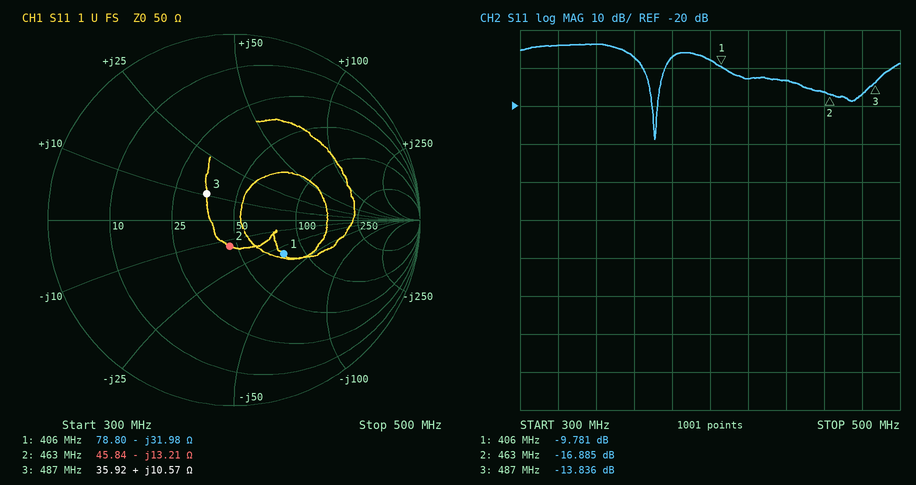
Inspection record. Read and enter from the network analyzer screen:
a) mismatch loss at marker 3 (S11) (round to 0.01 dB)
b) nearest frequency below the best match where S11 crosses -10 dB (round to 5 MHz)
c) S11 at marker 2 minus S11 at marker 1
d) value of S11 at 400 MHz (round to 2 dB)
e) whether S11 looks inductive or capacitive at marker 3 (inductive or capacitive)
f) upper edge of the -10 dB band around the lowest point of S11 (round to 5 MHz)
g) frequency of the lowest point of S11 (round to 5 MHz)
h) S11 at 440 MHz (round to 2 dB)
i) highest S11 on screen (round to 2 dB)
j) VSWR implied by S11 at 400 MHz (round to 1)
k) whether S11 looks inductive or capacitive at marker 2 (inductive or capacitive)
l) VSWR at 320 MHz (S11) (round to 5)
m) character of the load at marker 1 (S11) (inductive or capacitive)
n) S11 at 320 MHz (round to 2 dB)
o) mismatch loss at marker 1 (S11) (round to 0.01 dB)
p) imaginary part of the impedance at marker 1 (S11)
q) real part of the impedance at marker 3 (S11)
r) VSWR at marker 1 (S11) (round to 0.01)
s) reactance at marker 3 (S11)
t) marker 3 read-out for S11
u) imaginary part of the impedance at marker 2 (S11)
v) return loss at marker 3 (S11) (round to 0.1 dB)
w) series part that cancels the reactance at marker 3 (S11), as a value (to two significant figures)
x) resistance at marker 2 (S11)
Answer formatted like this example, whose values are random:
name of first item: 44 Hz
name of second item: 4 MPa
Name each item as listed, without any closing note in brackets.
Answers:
mismatch loss at marker 3 (S11): 0.18 dB
nearest frequency below the best match where S11 crosses -10 dB: 365 MHz
S11 at marker 2 minus S11 at marker 1: -7.104 dB
value of S11 at 400 MHz: -8 dB
whether S11 looks inductive or capacitive at marker 3: inductive
upper edge of the -10 dB band around the lowest point of S11: 375 MHz
frequency of the lowest point of S11: 370 MHz
S11 at 440 MHz: -14 dB
highest S11 on screen: -4 dB
VSWR implied by S11 at 400 MHz: 2
whether S11 looks inductive or capacitive at marker 2: capacitive
VSWR at 320 MHz (S11): 5
character of the load at marker 1 (S11): capacitive
S11 at 320 MHz: -4 dB
mismatch loss at marker 1 (S11): 0.48 dB
imaginary part of the impedance at marker 1: -31.98 Ω
real part of the impedance at marker 3: 35.92 Ω
VSWR at marker 1 (S11): 1.96
reactance at marker 3: +10.57 Ω
marker 3 read-out for S11: -13.836 dB
imaginary part of the impedance at marker 2: -13.21 Ω
return loss at marker 3 (S11): 13.8 dB
series part that cancels the reactance at marker 3 (S11), as a value: 31 pF
resistance at marker 2: 45.84 Ω
